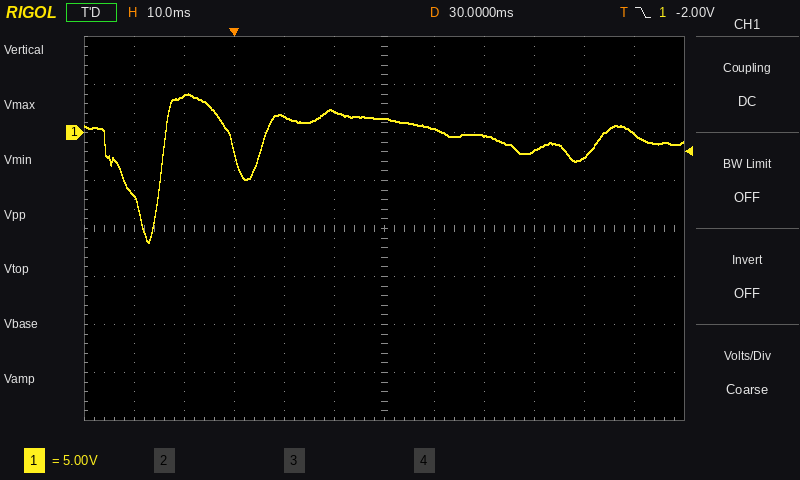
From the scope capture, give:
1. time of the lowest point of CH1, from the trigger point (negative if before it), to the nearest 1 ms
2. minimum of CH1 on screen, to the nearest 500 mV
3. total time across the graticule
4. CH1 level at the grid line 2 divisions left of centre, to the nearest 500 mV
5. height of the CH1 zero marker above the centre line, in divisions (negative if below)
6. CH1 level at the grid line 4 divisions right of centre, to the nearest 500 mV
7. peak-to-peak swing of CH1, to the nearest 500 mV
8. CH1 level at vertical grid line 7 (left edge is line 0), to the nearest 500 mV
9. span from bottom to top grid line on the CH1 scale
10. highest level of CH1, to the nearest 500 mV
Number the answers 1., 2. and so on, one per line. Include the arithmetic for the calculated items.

1. -17 ms
2. -11.5 V
3. 120 ms
4. 1.5 V
5. +2.0 div
6. -2.5 V
7. 4.0 V − (-11.5 V) = 15.5 V
8. 500 mV
9. 40 V
10. 4.0 V
